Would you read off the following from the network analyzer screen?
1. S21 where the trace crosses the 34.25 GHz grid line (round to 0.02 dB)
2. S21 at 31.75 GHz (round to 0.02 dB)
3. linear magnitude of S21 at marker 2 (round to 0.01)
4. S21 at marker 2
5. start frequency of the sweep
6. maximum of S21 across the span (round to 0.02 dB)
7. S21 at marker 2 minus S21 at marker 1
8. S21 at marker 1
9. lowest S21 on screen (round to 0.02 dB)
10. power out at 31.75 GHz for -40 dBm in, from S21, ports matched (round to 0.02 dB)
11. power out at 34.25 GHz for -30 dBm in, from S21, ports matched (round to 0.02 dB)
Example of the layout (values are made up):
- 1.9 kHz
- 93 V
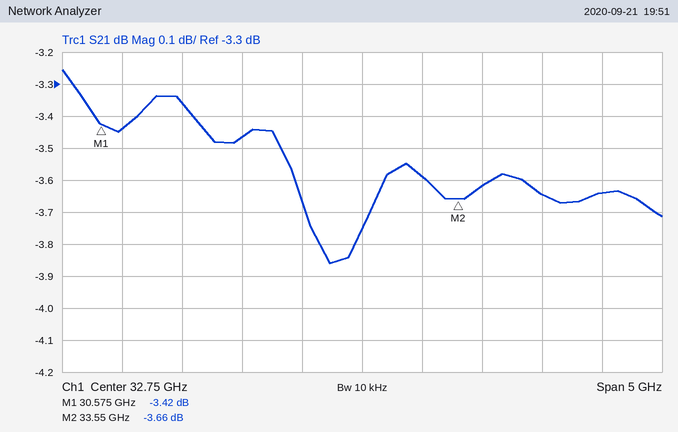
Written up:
- -3.64 dB
- -3.46 dB
- 0.66
- -3.66 dB
- 30.25 GHz
- -3.26 dB
- -0.24 dB
- -3.42 dB
- -3.86 dB
- -43.46 dBm
- -33.64 dBm
